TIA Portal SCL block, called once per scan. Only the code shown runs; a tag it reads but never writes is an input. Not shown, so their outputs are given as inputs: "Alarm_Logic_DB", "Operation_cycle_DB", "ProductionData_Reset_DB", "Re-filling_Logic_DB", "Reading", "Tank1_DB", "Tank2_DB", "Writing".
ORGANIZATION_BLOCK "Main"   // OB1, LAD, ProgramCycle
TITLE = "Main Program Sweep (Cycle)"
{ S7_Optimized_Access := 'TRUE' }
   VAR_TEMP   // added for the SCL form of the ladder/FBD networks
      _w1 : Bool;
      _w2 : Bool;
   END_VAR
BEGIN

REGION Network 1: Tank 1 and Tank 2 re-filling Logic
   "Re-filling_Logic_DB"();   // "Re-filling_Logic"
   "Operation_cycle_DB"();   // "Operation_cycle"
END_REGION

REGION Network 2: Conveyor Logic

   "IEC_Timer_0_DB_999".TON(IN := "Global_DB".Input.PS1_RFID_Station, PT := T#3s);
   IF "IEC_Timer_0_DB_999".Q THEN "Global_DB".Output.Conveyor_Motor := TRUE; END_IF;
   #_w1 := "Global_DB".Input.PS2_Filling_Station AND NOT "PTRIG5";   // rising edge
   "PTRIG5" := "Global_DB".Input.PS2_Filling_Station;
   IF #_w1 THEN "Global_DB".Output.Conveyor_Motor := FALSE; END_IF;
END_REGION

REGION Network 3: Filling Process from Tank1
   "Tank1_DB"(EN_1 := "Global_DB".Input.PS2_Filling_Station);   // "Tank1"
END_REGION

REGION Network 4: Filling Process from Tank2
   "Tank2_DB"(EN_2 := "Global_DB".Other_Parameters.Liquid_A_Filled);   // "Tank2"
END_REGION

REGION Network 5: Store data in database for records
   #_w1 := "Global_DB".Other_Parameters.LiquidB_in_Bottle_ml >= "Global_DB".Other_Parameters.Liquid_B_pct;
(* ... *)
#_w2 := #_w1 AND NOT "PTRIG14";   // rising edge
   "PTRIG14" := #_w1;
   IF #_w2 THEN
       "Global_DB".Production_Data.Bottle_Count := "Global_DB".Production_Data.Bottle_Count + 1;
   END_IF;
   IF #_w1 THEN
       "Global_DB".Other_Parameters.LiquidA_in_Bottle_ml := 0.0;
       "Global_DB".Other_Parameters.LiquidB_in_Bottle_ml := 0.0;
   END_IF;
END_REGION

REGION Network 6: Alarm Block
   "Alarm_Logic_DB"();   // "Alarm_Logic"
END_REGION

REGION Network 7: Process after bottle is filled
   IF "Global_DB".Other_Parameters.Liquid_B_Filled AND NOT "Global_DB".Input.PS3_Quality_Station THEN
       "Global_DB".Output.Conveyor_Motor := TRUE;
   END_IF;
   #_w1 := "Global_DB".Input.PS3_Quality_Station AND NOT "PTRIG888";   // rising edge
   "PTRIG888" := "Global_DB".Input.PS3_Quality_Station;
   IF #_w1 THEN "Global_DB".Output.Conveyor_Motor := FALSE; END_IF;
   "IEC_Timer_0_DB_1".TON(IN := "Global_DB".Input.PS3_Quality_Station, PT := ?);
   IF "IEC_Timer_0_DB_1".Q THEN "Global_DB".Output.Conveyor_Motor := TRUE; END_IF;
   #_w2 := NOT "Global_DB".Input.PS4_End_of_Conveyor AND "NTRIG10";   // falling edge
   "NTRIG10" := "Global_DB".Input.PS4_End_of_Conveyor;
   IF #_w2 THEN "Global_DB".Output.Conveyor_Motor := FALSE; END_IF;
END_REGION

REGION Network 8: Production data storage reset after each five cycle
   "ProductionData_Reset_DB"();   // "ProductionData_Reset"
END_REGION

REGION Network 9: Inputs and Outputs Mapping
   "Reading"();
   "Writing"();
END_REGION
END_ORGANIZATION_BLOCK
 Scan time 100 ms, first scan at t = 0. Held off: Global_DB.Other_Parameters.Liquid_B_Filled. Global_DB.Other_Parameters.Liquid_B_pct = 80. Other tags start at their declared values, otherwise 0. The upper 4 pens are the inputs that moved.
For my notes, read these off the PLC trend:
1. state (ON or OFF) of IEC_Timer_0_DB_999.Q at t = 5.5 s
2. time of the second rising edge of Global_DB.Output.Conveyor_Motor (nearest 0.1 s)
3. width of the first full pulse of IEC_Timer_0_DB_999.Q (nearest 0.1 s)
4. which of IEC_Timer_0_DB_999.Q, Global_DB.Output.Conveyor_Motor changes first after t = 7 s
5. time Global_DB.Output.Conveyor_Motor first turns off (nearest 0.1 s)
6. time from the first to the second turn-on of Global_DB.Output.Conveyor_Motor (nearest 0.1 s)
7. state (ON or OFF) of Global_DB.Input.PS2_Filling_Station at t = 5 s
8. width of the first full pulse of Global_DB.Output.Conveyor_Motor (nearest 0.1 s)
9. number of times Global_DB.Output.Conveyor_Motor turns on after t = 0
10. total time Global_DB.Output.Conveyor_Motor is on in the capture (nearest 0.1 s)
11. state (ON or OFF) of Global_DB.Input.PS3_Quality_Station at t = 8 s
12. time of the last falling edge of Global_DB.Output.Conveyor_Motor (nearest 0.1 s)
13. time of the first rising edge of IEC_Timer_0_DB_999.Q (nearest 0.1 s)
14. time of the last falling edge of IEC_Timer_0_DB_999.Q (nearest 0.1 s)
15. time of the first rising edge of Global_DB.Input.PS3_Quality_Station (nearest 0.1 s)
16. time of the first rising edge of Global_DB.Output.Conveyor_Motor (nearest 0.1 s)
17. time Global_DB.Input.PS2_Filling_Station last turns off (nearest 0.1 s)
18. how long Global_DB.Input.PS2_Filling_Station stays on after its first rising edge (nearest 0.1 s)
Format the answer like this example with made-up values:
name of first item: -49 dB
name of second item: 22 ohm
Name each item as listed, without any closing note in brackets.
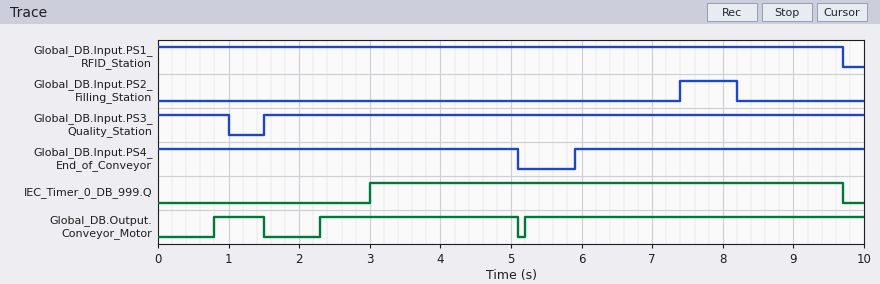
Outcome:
state (ON or OFF) of IEC_Timer_0_DB_999.Q at t = 5.5 s: ON
time of the second rising edge of Global_DB.Output.Conveyor_Motor: 2.3 s
width of the first full pulse of IEC_Timer_0_DB_999.Q: 6.7 s
which of IEC_Timer_0_DB_999.Q, Global_DB.Output.Conveyor_Motor changes first after t = 7 s: IEC_Timer_0_DB_999.Q
time Global_DB.Output.Conveyor_Motor first turns off: 1.5 s
time from the first to the second turn-on of Global_DB.Output.Conveyor_Motor: 1.5 s
state (ON or OFF) of Global_DB.Input.PS2_Filling_Station at t = 5 s: OFF
width of the first full pulse of Global_DB.Output.Conveyor_Motor: 0.7 s
number of times Global_DB.Output.Conveyor_Motor turns on after t = 0: 3
total time Global_DB.Output.Conveyor_Motor is on in the capture: 8.3 s
state (ON or OFF) of Global_DB.Input.PS3_Quality_Station at t = 8 s: ON
time of the last falling edge of Global_DB.Output.Conveyor_Motor: 5.1 s
time of the first rising edge of IEC_Timer_0_DB_999.Q: 3.0 s
time of the last falling edge of IEC_Timer_0_DB_999.Q: 9.7 s
time of the first rising edge of Global_DB.Input.PS3_Quality_Station: 1.5 s
time of the first rising edge of Global_DB.Output.Conveyor_Motor: 0.8 s
time Global_DB.Input.PS2_Filling_Station last turns off: 8.2 s
how long Global_DB.Input.PS2_Filling_Station stays on after its first rising edge: 0.8 s
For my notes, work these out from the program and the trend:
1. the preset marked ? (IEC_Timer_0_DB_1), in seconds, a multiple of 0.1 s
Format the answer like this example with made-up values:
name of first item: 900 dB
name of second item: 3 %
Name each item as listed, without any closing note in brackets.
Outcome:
the preset marked ? (IEC_Timer_0_DB_1), in seconds, a multiple of 0.1 s: 0.8 s
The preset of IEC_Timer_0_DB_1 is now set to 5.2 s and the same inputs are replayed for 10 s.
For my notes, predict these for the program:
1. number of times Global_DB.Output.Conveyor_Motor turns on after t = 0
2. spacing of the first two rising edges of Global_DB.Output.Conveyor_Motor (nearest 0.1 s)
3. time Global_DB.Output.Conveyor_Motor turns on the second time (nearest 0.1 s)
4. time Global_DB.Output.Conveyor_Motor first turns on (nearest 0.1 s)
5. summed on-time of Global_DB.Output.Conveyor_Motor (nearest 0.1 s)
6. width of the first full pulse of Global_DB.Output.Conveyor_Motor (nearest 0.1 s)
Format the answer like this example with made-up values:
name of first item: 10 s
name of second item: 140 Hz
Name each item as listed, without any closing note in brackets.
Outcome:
number of times Global_DB.Output.Conveyor_Motor turns on after t = 0: 2
spacing of the first two rising edges of Global_DB.Output.Conveyor_Motor: 2.2 s
time Global_DB.Output.Conveyor_Motor turns on the second time: 5.2 s
time Global_DB.Output.Conveyor_Motor first turns on: 3.0 s
summed on-time of Global_DB.Output.Conveyor_Motor: 6.9 s
width of the first full pulse of Global_DB.Output.Conveyor_Motor: 2.1 s
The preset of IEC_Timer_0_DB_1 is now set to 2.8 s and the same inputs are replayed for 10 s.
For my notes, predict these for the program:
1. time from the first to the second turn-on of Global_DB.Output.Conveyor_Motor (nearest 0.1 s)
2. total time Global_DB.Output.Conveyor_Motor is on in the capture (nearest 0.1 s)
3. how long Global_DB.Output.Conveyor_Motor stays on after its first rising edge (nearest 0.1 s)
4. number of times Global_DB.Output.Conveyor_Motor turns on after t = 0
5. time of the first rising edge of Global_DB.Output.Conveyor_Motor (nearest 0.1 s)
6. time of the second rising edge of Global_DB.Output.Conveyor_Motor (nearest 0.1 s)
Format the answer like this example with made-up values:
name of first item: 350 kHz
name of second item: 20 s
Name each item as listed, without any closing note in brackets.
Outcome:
time from the first to the second turn-on of Global_DB.Output.Conveyor_Motor: 2.2 s
total time Global_DB.Output.Conveyor_Motor is on in the capture: 6.9 s
how long Global_DB.Output.Conveyor_Motor stays on after its first rising edge: 2.1 s
number of times Global_DB.Output.Conveyor_Motor turns on after t = 0: 2
time of the first rising edge of Global_DB.Output.Conveyor_Motor: 3.0 s
time of the second rising edge of Global_DB.Output.Conveyor_Motor: 5.2 s
